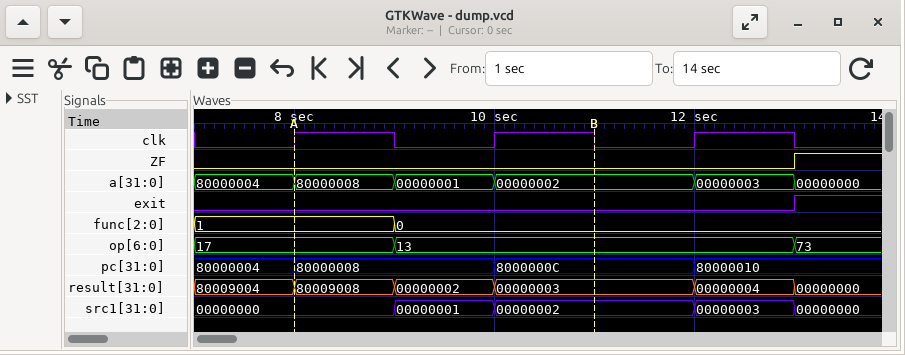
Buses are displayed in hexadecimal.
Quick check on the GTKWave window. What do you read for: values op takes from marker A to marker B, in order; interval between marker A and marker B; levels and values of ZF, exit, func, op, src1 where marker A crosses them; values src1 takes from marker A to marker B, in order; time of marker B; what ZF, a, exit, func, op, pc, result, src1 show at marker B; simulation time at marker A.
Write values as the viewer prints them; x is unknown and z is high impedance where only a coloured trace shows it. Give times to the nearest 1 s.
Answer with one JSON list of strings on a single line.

["17, 13", "3 s", "ZF=0, exit=0, func=1, op=17, src1=00000000", "00000000, 00000001, 00000002", "11 s", "ZF=0, a=00000002, exit=0, func=0, op=13, pc=8000000C, result=00000003, src1=00000002", "8 s"]
